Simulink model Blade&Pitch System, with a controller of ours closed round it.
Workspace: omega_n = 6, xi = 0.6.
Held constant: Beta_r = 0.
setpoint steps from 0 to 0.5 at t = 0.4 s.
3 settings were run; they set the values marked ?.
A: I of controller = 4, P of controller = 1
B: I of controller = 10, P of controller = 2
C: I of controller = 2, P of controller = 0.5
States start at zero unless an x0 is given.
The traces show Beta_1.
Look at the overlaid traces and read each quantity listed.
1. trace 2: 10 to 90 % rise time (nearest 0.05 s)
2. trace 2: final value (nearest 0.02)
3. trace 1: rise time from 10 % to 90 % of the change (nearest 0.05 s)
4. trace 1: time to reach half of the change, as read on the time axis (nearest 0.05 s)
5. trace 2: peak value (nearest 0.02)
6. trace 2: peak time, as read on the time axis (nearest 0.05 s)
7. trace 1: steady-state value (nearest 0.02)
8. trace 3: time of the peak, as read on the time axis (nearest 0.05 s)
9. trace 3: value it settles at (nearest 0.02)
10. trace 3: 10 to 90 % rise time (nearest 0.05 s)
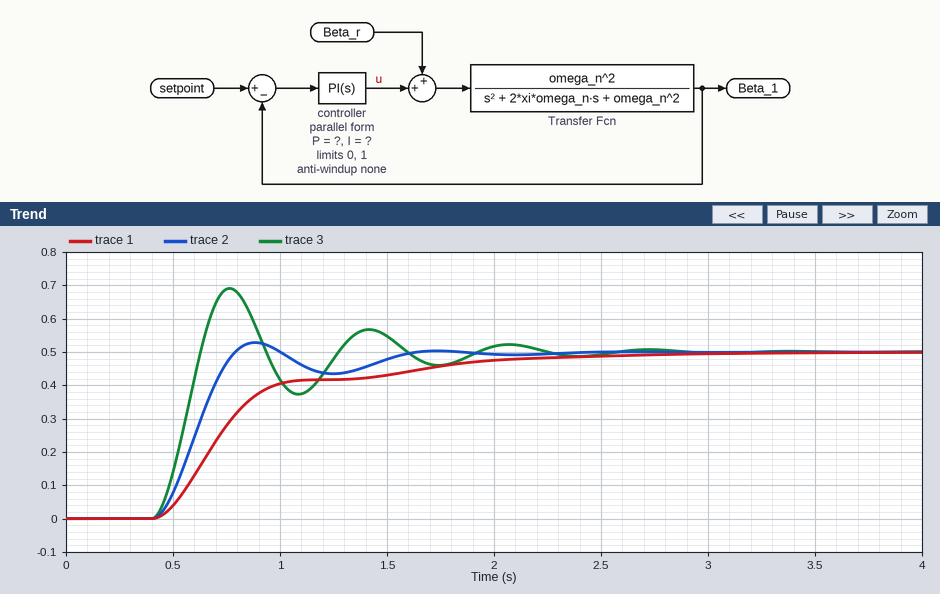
0.25 s
0.50
1.15 s
0.70 s
0.52
0.90 s
0.50
0.75 s
0.50
0.15 s
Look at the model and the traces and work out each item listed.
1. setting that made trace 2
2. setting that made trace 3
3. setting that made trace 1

A
B
C
